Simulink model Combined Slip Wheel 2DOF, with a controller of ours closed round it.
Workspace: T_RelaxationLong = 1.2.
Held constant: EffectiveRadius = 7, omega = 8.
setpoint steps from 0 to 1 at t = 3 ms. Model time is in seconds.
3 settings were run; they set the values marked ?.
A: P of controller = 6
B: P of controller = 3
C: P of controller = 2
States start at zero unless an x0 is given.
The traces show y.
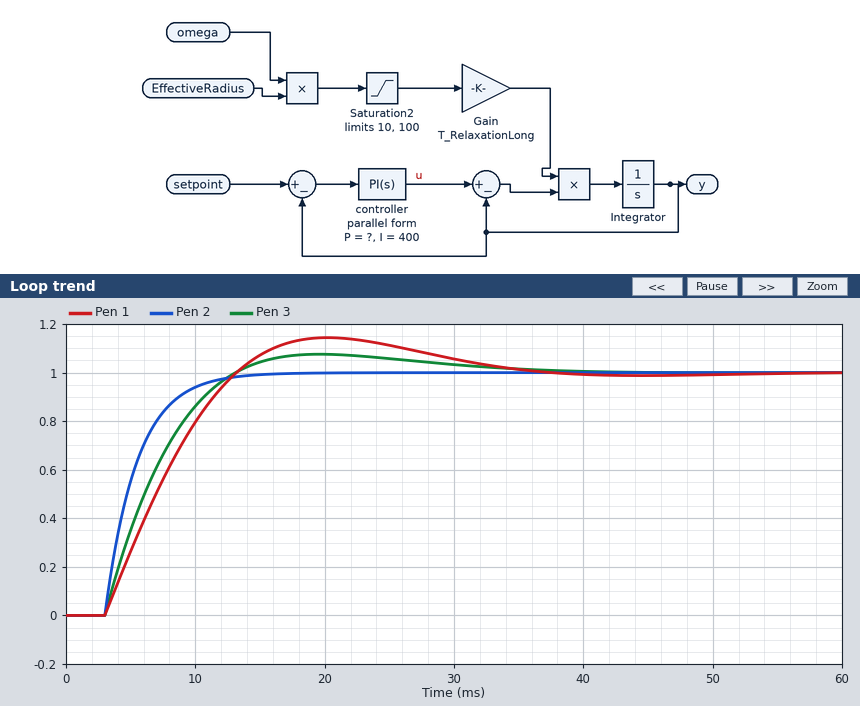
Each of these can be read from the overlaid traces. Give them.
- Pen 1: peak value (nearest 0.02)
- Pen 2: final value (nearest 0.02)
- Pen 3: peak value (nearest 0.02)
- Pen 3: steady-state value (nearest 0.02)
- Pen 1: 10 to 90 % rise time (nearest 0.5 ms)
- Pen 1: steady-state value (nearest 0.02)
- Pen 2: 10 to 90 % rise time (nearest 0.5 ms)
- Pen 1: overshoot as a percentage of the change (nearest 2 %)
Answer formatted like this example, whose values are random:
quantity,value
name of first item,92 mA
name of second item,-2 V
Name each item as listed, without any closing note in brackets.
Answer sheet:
quantity,value
Pen 1: peak value,1.14
Pen 2: final value,1.00
Pen 3: peak value,1.08
Pen 3: steady-state value,1.00
Pen 1: 10 to 90 % rise time,7.5 ms
Pen 1: steady-state value,1.00
Pen 2: 10 to 90 % rise time,5.5 ms
Pen 1: overshoot as a percentage of the change,14 %
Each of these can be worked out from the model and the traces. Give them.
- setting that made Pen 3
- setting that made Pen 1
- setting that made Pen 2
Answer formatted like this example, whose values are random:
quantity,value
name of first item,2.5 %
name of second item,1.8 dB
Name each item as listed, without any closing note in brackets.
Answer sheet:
quantity,value
setting that made Pen 3,B
setting that made Pen 1,C
setting that made Pen 2,A
